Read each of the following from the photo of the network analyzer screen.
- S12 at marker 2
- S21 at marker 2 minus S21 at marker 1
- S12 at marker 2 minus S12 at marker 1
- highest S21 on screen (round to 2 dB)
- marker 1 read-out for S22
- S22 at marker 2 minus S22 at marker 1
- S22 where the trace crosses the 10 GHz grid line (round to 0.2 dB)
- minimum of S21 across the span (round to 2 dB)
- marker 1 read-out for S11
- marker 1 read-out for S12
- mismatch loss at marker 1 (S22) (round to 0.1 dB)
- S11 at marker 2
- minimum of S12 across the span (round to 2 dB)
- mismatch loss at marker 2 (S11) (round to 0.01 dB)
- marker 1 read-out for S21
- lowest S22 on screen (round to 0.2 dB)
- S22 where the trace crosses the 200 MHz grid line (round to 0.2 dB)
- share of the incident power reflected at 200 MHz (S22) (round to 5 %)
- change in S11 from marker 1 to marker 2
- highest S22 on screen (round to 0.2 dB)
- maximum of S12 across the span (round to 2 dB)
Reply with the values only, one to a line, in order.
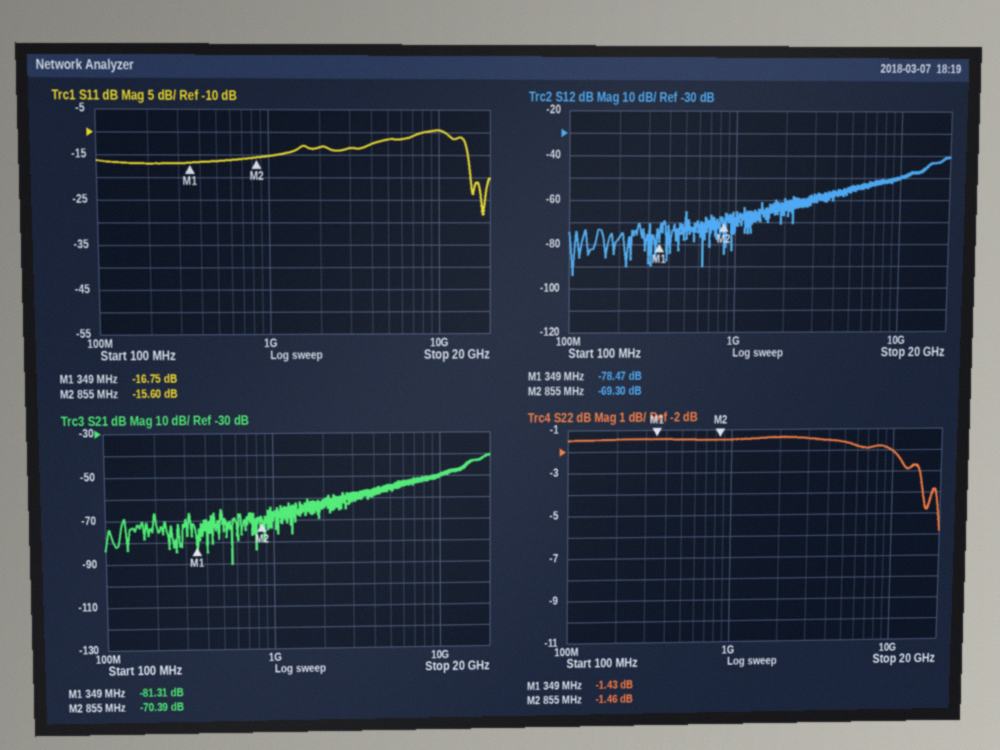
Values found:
-69.30 dB
10.92 dB
9.17 dB
-40 dB
-1.43 dB
-0.03 dB
-2.0 dB
-90 dB
-16.75 dB
-78.47 dB
5.5 dB
-15.60 dB
-94 dB
0.12 dB
-81.31 dB
-5.8 dB
-1.4 dB
70 %
1.15 dB
-1.4 dB
-40 dB
